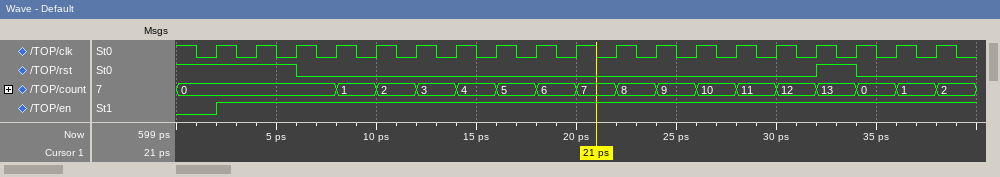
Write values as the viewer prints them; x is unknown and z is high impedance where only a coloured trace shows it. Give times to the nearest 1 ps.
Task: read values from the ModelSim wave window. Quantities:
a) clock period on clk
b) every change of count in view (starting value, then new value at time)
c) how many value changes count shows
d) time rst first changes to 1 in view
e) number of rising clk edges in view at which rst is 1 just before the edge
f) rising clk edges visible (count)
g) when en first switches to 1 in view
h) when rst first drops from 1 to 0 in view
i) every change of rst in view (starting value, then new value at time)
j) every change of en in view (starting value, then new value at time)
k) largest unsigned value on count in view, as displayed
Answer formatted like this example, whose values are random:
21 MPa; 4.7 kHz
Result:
2 ps; 0, 1 at 8 ps, 2 at 10 ps, 3 at 12 ps, 4 at 14 ps, 5 at 16 ps, 6 at 18 ps, 7 at 20 ps, 8 at 22 ps, 9 at 24 ps, 10 at 26 ps, 11 at 28 ps, 12 at 30 ps, 13 at 32 ps, 0 at 34 ps, 1 at 36 ps, 2 at 38 ps; 16; 32 ps; 4; 19; 2 ps; 6 ps; 1, 0 at 6 ps, 1 at 32 ps, 0 at 34 ps; 0, 1 at 2 ps; 13
